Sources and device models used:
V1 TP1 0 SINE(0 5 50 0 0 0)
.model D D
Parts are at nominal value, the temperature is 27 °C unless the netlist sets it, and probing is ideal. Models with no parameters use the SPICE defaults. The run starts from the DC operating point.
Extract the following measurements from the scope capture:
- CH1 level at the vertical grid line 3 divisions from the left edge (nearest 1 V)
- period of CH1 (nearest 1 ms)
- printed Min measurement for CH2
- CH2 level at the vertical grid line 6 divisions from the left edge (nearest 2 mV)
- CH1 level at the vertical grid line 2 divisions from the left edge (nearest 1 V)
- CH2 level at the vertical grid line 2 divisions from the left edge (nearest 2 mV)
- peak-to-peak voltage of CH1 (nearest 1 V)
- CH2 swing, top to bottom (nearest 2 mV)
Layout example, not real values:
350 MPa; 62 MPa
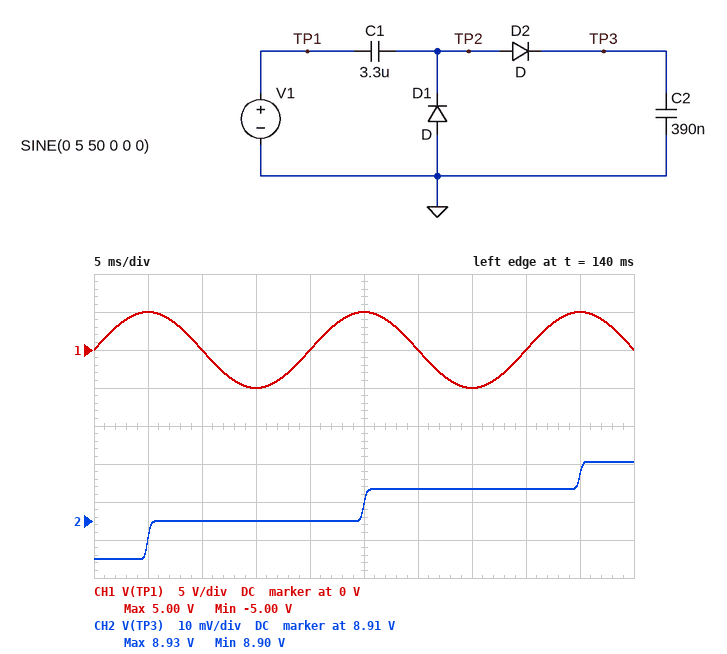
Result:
-5 V; 20 ms; 8.90 V; 8.918 V; 0 V; 8.910 V; 10 V; 26 mV
